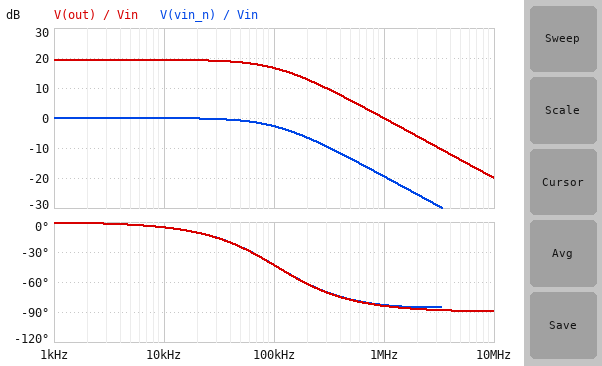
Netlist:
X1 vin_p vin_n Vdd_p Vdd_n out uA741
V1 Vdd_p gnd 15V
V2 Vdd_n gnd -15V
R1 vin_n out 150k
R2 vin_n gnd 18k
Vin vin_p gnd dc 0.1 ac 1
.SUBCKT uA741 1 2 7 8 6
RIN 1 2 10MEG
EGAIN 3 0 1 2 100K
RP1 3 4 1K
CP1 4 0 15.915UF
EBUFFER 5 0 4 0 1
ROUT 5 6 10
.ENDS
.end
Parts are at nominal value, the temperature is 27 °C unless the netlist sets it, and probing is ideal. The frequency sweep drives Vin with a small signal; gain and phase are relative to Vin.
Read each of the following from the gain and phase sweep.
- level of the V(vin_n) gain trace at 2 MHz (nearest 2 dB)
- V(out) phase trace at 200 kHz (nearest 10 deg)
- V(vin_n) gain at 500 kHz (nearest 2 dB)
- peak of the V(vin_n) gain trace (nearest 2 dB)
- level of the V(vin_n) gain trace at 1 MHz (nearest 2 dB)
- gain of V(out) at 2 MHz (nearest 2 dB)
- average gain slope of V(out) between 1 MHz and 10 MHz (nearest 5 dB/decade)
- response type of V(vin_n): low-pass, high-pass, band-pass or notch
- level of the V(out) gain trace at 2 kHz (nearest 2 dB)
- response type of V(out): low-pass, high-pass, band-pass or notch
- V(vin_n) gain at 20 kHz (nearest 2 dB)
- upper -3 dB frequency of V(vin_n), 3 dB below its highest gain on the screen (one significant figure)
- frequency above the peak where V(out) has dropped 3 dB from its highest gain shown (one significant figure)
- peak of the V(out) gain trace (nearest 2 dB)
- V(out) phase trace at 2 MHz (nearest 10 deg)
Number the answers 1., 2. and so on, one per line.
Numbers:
1. -26 dB
2. -60 deg
3. -14 dB
4. 0 dB
5. -20 dB
6. -6 dB
7. -20 dB/decade
8. low-pass
9. 20 dB
10. low-pass
11. 0 dB
12. 100 kHz
13. 100 kHz
14. 20 dB
15. -90 deg
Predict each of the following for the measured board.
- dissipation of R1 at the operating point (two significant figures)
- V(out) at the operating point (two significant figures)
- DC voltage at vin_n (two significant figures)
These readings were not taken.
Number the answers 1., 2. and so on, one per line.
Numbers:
1. 4.6 µW
2. 930 mV
3. 100 mV
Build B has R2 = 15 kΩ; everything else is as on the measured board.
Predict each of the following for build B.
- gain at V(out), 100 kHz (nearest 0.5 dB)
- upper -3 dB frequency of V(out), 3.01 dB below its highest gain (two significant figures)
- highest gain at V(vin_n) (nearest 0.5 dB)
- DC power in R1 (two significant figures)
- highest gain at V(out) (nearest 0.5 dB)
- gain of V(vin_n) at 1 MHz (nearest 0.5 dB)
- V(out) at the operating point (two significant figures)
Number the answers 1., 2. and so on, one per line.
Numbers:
1. 17.5 dB
2. 91 kHz
3. 0 dB
4. 6.7 µW
5. 21.0 dB
6. -21.0 dB
7. 1.1 V
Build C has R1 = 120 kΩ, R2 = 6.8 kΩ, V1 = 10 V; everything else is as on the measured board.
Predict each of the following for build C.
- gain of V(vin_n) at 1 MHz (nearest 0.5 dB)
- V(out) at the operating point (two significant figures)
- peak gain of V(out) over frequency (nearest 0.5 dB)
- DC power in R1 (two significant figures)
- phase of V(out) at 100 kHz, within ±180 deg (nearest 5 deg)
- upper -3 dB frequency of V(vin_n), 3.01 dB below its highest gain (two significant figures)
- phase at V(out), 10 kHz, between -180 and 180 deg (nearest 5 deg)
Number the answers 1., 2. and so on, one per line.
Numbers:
1. -25.5 dB
2. 1.9 V
3. 25.5 dB
4. 26 µW
5. -60 deg
6. 54 kHz
7. -10 deg
